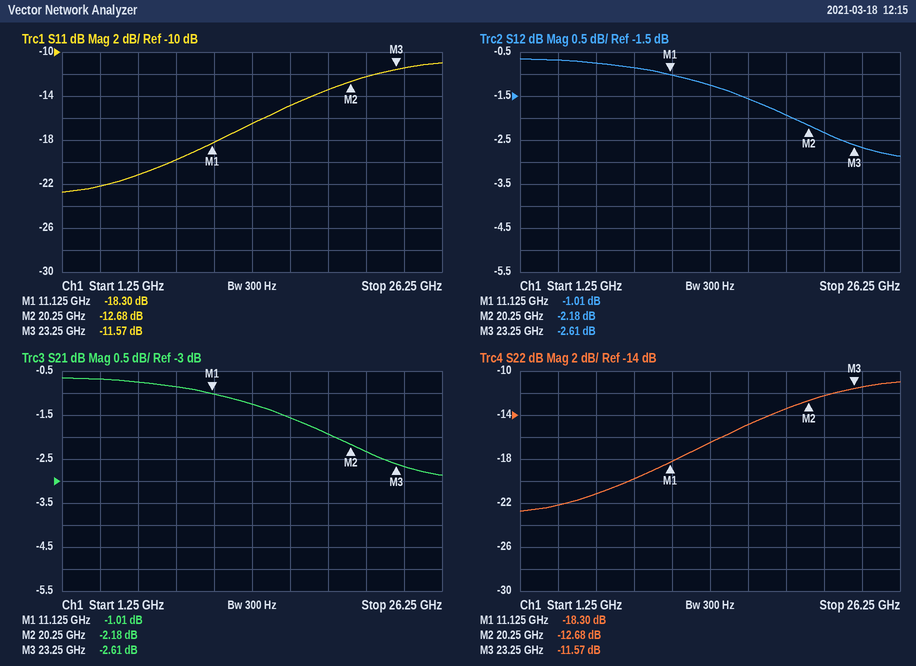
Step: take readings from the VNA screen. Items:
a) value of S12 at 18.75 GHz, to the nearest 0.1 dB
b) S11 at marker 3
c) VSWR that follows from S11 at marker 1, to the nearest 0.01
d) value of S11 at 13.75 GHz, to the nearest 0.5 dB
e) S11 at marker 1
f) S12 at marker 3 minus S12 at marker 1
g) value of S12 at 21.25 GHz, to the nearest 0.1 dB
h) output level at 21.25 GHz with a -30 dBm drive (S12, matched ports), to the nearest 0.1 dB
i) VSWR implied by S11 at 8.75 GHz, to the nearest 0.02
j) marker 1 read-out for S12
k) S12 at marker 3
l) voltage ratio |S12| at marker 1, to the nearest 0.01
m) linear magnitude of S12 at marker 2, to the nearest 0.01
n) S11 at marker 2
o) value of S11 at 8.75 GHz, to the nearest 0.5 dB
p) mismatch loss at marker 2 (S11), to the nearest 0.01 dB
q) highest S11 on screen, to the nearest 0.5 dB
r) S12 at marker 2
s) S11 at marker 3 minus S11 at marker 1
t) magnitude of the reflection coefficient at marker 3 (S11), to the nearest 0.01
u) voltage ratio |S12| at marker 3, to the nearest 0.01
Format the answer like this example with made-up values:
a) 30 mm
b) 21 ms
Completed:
a) -1.9 dB
b) -11.57 dB
c) 1.28
d) -16.5 dB
e) -18.30 dB
f) -1.60 dB
g) -2.3 dB
h) -32.3 dBm
i) 1.22
j) -1.01 dB
k) -2.61 dB
l) 0.89
m) 0.78
n) -12.68 dB
o) -20.0 dB
p) 0.24 dB
q) -11.0 dB
r) -2.18 dB
s) 6.73 dB
t) 0.26
u) 0.74
